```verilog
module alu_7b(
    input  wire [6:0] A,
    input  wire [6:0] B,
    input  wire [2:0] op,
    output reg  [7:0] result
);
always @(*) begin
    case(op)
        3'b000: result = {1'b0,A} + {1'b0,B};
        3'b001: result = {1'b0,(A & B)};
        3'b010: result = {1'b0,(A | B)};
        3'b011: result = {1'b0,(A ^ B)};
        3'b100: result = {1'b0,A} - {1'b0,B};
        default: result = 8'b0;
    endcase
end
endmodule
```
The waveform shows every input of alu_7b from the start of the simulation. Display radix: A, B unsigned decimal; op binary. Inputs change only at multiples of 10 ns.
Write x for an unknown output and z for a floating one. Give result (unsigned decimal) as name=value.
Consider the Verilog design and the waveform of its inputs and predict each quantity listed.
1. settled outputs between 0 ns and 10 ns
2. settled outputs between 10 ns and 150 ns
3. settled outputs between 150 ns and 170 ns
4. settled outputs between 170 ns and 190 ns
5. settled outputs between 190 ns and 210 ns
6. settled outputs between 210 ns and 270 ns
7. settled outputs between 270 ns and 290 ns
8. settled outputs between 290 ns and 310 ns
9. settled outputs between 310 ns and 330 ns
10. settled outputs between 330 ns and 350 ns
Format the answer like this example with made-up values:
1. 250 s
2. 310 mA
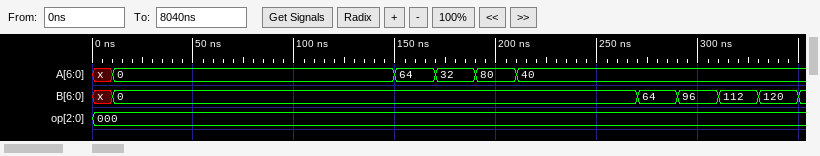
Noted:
1. result=x
2. result=0
3. result=64
4. result=32
5. result=80
6. result=40
7. result=104
8. result=136
9. result=152
10. result=160
